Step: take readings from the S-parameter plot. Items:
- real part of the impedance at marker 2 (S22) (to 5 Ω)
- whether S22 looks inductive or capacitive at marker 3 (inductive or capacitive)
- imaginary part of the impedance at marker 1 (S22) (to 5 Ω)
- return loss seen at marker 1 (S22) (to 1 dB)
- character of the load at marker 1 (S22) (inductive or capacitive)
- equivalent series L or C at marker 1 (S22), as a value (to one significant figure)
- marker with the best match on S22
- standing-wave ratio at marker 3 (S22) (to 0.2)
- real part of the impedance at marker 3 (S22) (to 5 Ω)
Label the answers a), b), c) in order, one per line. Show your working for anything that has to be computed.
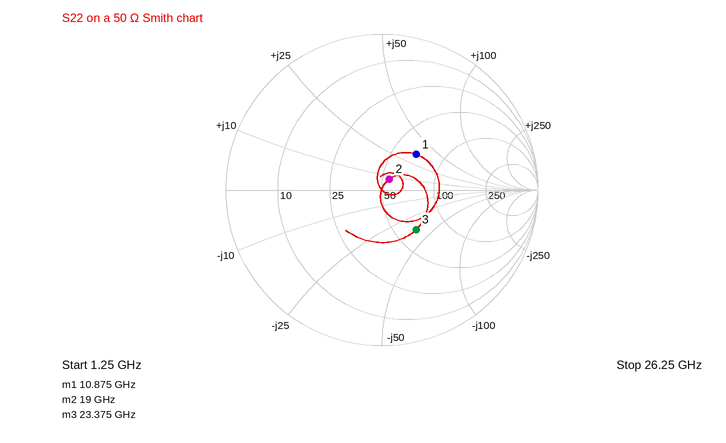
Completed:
a) 55 Ω
b) capacitive
c) +35 Ω
d) 10 dB
e) inductive
f) L = 35 Ω/(2π × 10.875 GHz) ≈ 512 pH, so 500 pH to one significant figure
g) marker 2
h) 2.0
i) 65 Ω
